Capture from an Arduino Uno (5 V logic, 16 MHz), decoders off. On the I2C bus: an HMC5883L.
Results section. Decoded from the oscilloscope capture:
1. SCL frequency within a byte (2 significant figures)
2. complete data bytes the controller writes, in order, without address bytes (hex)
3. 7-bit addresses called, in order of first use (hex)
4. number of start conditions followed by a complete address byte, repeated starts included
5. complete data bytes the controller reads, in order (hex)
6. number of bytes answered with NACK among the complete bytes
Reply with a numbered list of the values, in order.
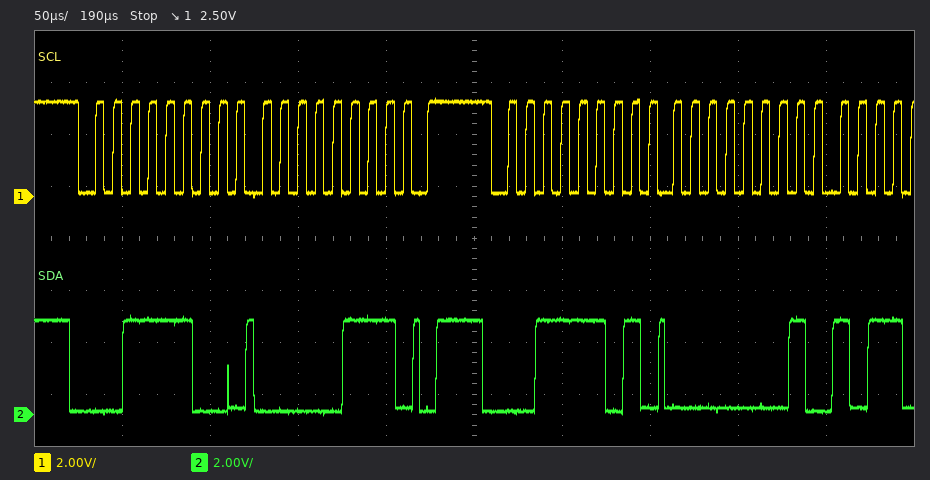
1. 100 kHz
2. 07
3. 0x1E
4. 2
5. 01
6. 0
